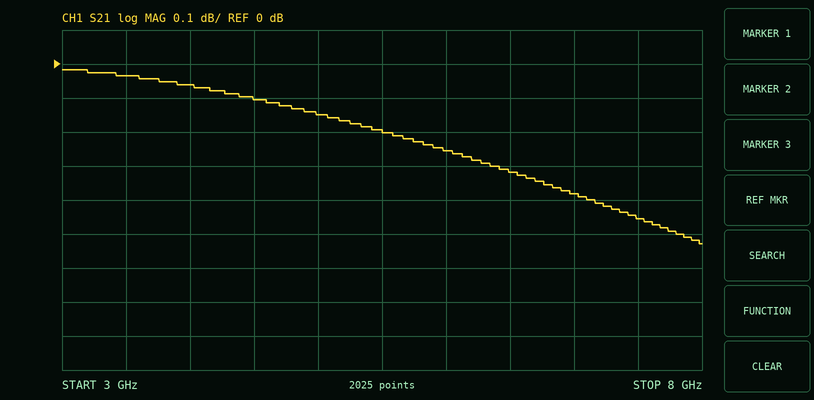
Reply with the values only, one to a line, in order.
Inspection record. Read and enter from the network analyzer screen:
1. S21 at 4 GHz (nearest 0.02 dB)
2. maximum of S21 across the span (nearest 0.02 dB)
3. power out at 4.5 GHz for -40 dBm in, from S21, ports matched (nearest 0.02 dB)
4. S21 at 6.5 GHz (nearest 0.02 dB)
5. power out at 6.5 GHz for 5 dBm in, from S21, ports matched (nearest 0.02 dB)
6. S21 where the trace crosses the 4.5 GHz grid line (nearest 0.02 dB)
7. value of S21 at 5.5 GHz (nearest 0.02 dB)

-0.06 dB
-0.02 dB
-40.10 dBm
-0.32 dB
4.68 dBm
-0.10 dB
-0.20 dB
